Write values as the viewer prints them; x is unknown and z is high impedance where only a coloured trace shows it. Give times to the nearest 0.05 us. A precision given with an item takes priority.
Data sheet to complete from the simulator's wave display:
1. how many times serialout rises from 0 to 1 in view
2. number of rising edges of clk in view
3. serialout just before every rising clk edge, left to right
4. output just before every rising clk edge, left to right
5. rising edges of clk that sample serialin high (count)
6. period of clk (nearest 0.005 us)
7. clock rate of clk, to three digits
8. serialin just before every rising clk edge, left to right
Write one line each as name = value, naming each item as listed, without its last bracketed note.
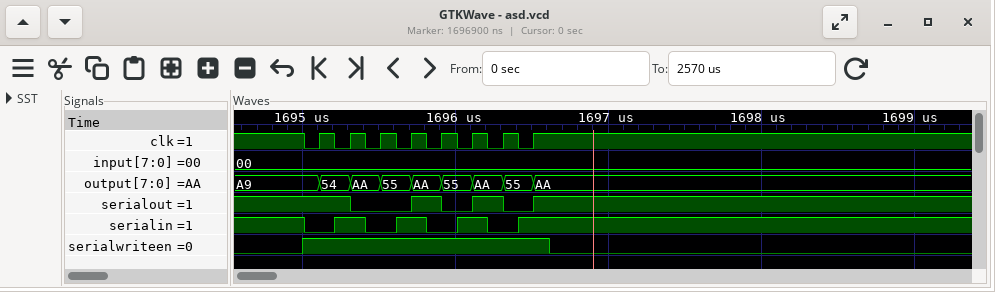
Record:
how many times serialout rises from 0 to 1 in view = 3
number of rising edges of clk in view = 8
serialout just before every rising clk edge, left to right = 1 1 0 0 1 0 1 0
output just before every rising clk edge, left to right = A9, 54, AA, 55, AA, 55, AA, 55
rising edges of clk that sample serialin high = 4
period of clk = 0.2 us
clock rate of clk, to three digits = 5.00 MHz
serialin just before every rising clk edge, left to right = 0 1 0 1 0 1 0 1
